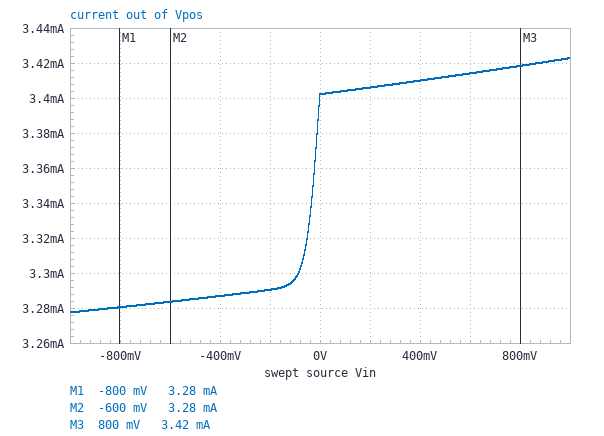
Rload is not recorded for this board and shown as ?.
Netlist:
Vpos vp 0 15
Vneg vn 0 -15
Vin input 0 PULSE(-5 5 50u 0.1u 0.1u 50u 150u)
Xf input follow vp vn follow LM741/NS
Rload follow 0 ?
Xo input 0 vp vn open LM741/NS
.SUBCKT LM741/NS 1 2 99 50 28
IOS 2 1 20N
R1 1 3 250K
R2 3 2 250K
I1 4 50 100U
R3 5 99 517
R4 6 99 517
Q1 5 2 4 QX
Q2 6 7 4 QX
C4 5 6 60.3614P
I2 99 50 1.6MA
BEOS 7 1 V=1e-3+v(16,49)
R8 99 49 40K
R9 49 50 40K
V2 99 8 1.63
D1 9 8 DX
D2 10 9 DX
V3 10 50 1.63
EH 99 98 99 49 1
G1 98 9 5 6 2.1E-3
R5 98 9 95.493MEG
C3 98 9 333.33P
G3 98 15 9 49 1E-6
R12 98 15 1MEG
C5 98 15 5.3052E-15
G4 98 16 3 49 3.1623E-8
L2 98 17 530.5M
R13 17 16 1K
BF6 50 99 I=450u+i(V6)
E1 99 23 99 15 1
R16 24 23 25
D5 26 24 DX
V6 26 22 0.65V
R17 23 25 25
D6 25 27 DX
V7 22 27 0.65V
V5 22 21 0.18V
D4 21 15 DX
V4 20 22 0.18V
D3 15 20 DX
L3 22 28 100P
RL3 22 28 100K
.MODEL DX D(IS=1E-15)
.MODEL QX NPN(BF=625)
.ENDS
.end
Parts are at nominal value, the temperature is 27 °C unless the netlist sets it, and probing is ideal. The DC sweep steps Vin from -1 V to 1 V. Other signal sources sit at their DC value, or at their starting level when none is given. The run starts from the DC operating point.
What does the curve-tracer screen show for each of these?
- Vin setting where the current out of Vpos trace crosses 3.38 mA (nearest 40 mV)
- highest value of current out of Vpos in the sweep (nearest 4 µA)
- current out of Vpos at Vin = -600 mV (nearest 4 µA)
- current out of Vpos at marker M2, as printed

0 V
3.424 mA
3.284 mA
3.28 mA
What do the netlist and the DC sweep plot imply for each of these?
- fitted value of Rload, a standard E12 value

27 kΩ
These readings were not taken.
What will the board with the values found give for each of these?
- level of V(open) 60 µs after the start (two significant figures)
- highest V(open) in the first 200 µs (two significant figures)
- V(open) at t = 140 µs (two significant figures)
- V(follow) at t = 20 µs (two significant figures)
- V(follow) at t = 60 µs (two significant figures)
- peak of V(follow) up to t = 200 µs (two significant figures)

-11 V
2.3 V
-11 V
-5.0 V
-1.8 V
5.0 V
